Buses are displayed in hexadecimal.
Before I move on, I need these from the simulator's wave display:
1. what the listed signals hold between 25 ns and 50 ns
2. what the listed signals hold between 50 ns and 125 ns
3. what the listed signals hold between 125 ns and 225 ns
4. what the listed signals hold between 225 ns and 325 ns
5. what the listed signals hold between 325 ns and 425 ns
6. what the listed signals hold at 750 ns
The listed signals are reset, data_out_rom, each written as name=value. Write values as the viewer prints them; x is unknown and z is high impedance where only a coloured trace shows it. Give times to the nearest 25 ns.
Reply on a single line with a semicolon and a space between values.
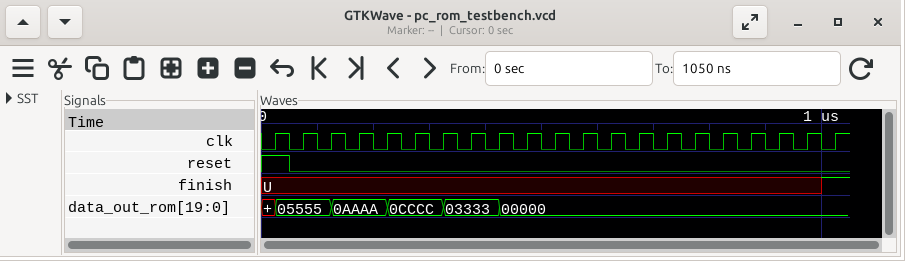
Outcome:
reset=1, data_out_rom=05555; reset=0, data_out_rom=05555; reset=0, data_out_rom=0AAAA; reset=0, data_out_rom=0CCCC; reset=0, data_out_rom=03333; reset=0, data_out_rom=00000
